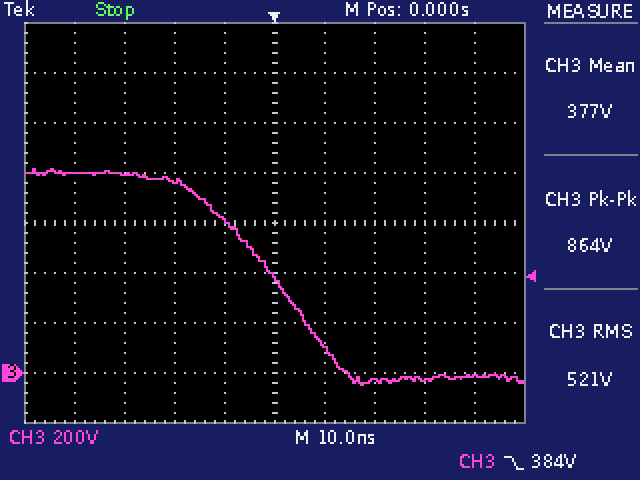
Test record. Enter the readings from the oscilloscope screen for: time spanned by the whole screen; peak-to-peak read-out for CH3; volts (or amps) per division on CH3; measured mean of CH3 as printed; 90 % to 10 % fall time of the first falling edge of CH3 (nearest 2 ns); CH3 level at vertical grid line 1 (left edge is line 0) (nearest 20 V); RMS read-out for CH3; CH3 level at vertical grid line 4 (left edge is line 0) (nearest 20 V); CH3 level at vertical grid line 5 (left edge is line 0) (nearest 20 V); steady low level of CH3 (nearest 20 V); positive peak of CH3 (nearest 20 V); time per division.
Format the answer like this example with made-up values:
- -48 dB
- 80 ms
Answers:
- 100 ns
- 864 V
- 200 V
- 377 V
- 28 ns
- 800 V
- 521 V
- 620 V
- 380 V
- -20 V
- 820 V
- 10 ns
